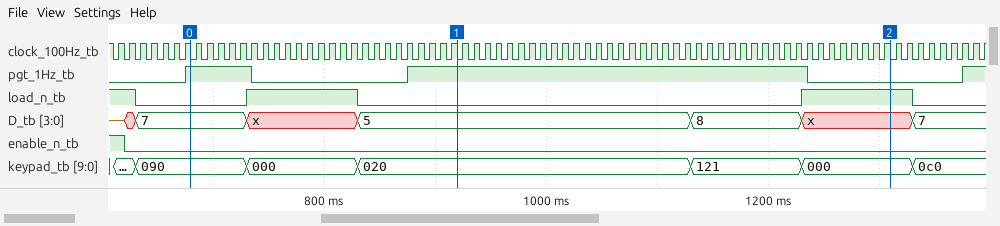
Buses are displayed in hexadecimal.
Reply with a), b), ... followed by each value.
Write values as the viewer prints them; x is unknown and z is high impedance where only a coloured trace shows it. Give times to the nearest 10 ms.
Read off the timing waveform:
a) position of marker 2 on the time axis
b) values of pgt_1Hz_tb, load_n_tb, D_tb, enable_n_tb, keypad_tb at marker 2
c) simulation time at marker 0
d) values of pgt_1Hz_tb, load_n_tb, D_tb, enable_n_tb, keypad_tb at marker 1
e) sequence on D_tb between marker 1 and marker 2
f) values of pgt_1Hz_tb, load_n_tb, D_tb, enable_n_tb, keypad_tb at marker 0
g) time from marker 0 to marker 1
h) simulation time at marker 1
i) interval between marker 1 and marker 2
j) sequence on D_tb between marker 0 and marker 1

a) 1310 ms
b) pgt_1Hz_tb=0, load_n_tb=1, D_tb=x, enable_n_tb=0, keypad_tb=000
c) 680 ms
d) pgt_1Hz_tb=1, load_n_tb=0, D_tb=5, enable_n_tb=0, keypad_tb=020
e) 5, 8, x
f) pgt_1Hz_tb=1, load_n_tb=0, D_tb=7, enable_n_tb=0, keypad_tb=090
g) 240 ms
h) 920 ms
i) 390 ms
j) 7, x, 5
